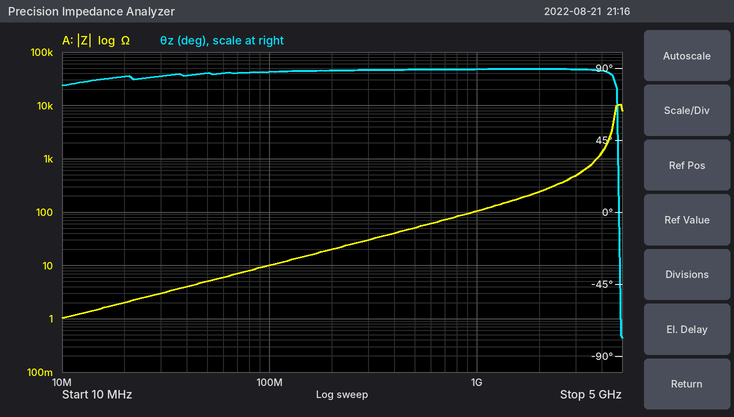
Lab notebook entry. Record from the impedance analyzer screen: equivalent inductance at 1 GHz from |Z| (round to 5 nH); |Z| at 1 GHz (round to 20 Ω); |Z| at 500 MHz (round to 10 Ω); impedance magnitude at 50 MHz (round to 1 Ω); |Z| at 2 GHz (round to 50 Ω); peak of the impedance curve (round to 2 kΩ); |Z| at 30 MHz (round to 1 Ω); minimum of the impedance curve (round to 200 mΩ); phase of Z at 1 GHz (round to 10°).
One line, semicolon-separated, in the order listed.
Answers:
15 nH; 100 Ω; 50 Ω; 5 Ω; 250 Ω; 10 kΩ; 3 Ω; 1.0 Ω; 90°
